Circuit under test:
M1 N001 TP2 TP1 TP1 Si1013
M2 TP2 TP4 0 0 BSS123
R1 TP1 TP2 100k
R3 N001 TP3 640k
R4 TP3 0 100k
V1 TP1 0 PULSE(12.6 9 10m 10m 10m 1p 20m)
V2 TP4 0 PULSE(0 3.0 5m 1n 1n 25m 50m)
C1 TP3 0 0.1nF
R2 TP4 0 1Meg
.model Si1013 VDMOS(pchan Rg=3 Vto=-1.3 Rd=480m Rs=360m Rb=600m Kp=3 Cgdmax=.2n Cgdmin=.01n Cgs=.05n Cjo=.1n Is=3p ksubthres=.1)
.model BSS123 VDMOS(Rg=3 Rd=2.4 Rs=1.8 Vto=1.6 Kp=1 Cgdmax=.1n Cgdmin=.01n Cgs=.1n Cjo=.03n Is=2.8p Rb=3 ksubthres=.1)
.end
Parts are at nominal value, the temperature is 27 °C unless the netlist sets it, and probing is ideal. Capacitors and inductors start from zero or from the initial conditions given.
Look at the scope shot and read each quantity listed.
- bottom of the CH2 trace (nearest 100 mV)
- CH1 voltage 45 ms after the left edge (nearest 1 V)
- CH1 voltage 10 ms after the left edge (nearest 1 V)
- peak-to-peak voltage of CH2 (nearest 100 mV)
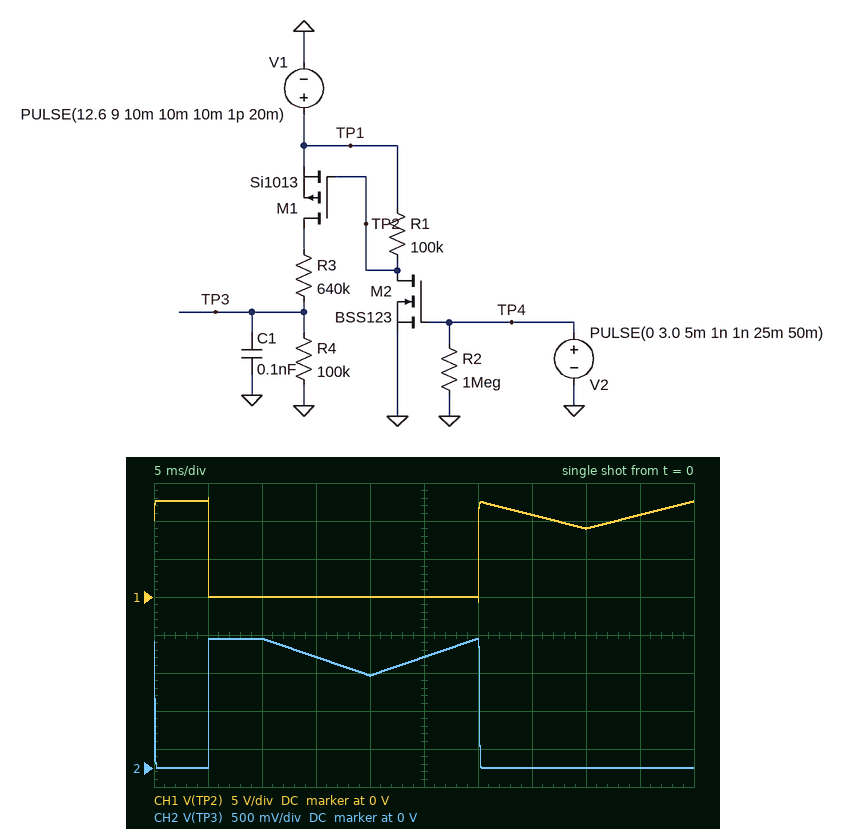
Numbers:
0 V
11 V
0 V
1.7 V
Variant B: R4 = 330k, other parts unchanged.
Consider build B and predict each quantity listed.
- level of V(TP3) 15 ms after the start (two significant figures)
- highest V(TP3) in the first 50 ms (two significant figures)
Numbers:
3.7 V
4.3 V
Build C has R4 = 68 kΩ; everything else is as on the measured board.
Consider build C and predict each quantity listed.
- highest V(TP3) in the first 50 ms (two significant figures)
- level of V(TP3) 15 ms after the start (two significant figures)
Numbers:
1.2 V
1.0 V
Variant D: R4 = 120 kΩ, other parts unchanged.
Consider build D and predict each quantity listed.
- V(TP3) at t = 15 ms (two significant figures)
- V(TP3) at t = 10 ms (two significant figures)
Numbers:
1.7 V
2.0 V
